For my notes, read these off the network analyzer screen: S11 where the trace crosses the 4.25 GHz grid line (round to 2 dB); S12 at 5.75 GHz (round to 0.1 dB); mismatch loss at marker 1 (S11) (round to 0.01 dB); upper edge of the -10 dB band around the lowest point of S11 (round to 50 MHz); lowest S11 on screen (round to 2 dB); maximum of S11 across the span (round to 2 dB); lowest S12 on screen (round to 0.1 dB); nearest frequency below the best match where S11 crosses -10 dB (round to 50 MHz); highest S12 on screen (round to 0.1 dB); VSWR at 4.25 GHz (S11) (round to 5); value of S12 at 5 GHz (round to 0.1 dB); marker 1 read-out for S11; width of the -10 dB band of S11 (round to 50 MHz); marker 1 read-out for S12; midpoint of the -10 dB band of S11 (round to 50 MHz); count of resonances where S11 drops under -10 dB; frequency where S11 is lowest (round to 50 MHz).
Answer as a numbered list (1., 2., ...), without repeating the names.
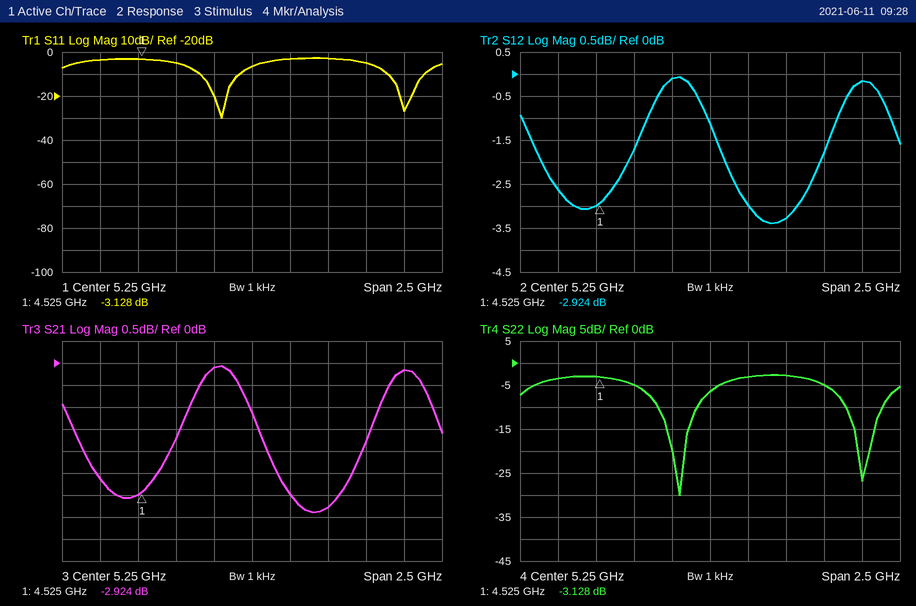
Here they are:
1. -4 dB
2. -3.3 dB
3. 2.90 dB
4. 5.15 GHz
5. -30 dB
6. -2 dB
7. -3.4 dB
8. 4.90 GHz
9. -0.1 dB
10. 5
11. -0.1 dB
12. -3.128 dB
13. 250 MHz
14. -2.924 dB
15. 5.05 GHz
16. 2
17. 5.05 GHz
